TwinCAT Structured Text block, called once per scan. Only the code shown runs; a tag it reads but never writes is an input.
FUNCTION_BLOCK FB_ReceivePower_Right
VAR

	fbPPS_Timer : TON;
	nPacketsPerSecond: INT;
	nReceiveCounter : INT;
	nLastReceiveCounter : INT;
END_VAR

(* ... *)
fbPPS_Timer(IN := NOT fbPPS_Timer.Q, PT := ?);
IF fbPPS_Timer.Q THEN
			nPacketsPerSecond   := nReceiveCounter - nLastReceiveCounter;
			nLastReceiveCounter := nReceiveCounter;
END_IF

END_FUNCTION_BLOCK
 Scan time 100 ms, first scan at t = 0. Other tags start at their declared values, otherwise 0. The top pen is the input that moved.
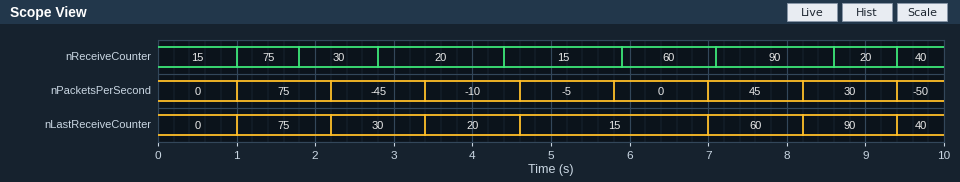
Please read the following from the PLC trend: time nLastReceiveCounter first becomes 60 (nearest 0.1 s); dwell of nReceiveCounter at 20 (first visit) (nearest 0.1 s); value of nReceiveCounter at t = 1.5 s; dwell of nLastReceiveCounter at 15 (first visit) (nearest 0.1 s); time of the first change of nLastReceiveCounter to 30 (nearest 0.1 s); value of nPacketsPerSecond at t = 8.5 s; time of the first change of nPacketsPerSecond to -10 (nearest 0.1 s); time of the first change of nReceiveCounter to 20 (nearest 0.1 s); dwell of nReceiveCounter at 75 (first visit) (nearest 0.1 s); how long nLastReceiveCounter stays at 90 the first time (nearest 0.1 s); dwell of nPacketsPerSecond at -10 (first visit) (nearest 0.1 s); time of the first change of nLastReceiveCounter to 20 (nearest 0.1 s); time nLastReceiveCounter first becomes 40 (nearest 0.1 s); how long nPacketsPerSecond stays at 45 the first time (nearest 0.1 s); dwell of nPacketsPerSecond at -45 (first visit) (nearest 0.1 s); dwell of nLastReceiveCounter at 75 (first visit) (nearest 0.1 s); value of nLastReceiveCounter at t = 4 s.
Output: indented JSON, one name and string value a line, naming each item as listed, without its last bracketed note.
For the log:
{
  "time nLastReceiveCounter first becomes 60": "7.0 s",
  "dwell of nReceiveCounter at 20 (first visit)": "1.6 s",
  "value of nReceiveCounter at t = 1.5 s": "75",
  "dwell of nLastReceiveCounter at 15 (first visit)": "2.4 s",
  "time of the first change of nLastReceiveCounter to 30": "2.2 s",
  "value of nPacketsPerSecond at t = 8.5 s": "30",
  "time of the first change of nPacketsPerSecond to -10": "3.4 s",
  "time of the first change of nReceiveCounter to 20": "2.8 s",
  "dwell of nReceiveCounter at 75 (first visit)": "0.8 s",
  "how long nLastReceiveCounter stays at 90 the first time": "1.2 s",
  "dwell of nPacketsPerSecond at -10 (first visit)": "1.2 s",
  "time of the first change of nLastReceiveCounter to 20": "3.4 s",
  "time nLastReceiveCounter first becomes 40": "9.4 s",
  "how long nPacketsPerSecond stays at 45 the first time": "1.2 s",
  "dwell of nPacketsPerSecond at -45 (first visit)": "1.2 s",
  "dwell of nLastReceiveCounter at 75 (first visit)": "1.2 s",
  "value of nLastReceiveCounter at t = 4 s": "20"
}
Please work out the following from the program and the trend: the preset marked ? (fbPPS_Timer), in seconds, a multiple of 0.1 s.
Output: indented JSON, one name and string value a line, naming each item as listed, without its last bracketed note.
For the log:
{
  "the preset marked ? (fbPPS_Timer), in seconds, a multiple of 0.1 s": "1.0 s"
}
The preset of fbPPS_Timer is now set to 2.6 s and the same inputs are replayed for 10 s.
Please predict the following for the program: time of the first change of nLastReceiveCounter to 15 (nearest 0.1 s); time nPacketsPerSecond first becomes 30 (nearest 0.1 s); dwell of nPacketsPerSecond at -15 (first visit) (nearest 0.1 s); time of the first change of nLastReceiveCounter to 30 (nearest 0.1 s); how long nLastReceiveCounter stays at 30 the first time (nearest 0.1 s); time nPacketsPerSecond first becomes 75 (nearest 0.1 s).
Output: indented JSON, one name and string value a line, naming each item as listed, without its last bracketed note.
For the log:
{
  "time of the first change of nLastReceiveCounter to 15": "5.4 s",
  "time nPacketsPerSecond first becomes 30": "2.6 s",
  "dwell of nPacketsPerSecond at -15 (first visit)": "2.8 s",
  "time of the first change of nLastReceiveCounter to 30": "2.6 s",
  "how long nLastReceiveCounter stays at 30 the first time": "2.8 s",
  "time nPacketsPerSecond first becomes 75": "8.2 s"
}
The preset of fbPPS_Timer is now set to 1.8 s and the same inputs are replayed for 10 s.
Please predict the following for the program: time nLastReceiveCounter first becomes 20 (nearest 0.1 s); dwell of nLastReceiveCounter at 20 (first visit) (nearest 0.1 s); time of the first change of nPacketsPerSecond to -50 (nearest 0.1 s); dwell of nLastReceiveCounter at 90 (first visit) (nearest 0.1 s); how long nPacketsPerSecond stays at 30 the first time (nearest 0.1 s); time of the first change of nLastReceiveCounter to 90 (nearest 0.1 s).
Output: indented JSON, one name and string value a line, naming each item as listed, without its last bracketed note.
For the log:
{
  "time nLastReceiveCounter first becomes 20": "3.8 s",
  "dwell of nLastReceiveCounter at 20 (first visit)": "2.0 s",
  "time of the first change of nPacketsPerSecond to -50": "9.8 s",
  "dwell of nLastReceiveCounter at 90 (first visit)": "2.0 s",
  "how long nPacketsPerSecond stays at 30 the first time": "2.0 s",
  "time of the first change of nLastReceiveCounter to 90": "7.8 s"
}
